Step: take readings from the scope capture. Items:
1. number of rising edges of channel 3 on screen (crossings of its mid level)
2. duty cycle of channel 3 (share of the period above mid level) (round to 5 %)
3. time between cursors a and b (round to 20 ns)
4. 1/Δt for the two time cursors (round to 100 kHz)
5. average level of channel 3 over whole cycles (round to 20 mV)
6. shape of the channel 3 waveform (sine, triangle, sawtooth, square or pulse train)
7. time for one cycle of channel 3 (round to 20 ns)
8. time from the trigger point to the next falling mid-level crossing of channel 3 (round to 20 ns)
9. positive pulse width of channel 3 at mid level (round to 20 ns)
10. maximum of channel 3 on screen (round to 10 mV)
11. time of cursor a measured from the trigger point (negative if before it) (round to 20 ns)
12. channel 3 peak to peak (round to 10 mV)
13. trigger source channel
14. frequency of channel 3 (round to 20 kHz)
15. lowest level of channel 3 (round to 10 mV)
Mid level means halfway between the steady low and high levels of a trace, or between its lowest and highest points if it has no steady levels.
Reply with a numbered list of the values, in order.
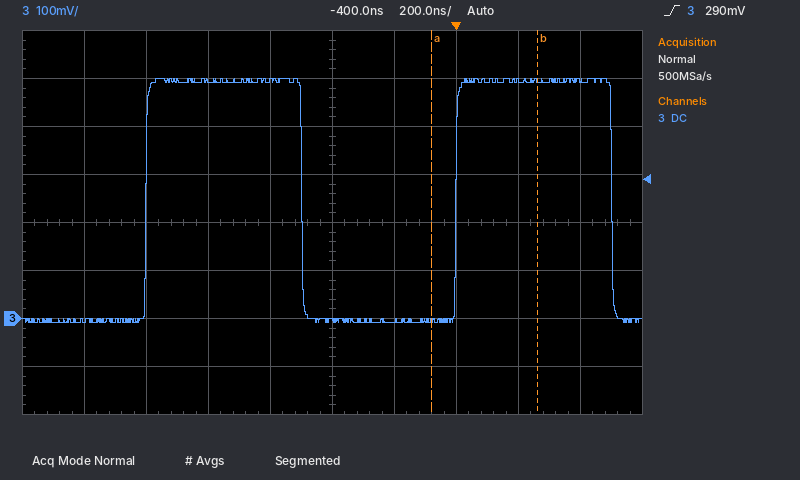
1. 2
2. 50 %
3. 340 ns
4. 2.9 MHz
5. 240 mV
6. square
7. 1.00 µs
8. 500 ns
9. 500 ns
10. 500 mV
11. -80 ns
12. 510 mV
13. channel 3
14. 1.00 MHz
15. -10 mV
